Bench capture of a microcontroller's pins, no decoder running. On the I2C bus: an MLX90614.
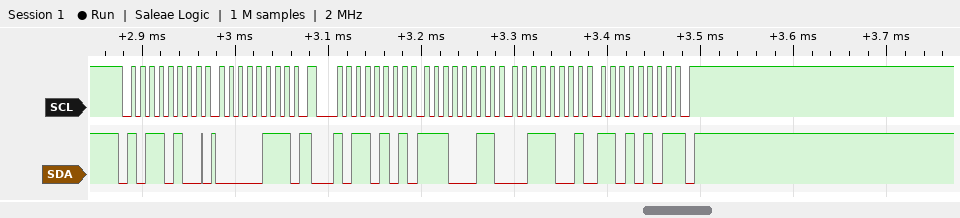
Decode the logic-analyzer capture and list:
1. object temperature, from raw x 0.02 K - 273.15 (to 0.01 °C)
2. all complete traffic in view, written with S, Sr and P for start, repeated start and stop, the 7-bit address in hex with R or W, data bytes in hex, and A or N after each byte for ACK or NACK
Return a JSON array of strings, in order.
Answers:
["23.23 °C", "S 5AW A 07 A Sr 5AR A E3 A 39 A D5 N P"]
